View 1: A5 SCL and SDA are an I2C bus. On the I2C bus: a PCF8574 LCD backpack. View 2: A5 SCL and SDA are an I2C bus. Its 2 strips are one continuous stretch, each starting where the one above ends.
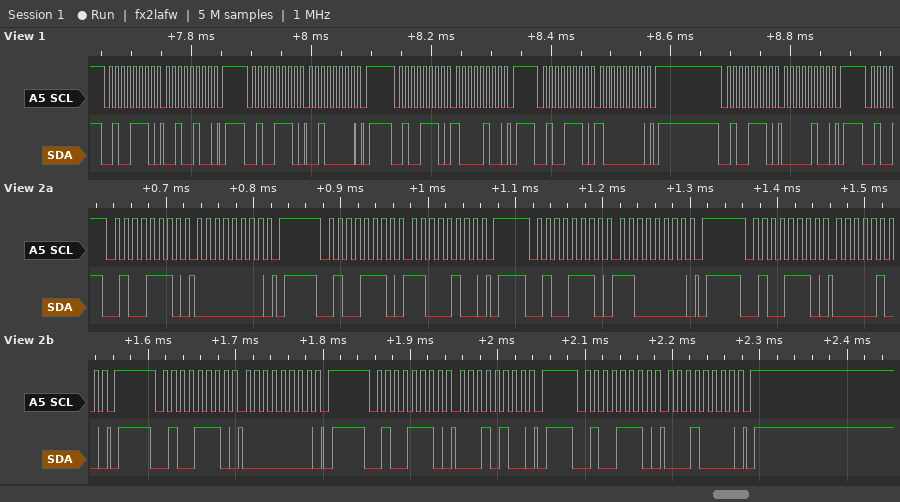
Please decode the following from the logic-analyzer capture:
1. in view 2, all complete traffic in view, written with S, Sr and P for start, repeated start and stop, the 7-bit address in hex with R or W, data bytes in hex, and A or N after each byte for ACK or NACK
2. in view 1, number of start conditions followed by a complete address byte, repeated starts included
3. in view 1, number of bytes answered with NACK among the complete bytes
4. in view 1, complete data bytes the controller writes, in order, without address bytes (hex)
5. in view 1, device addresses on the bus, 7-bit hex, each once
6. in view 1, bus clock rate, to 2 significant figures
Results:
S 27W A 00 A P S 27W A C4 A P S 27W A C0 A P S 27W A 04 A P S 27W A 00 A P S 27W A 14 A P S 27W A 10 A P
5
0
24 20 84 80 04
0x27
100 kHz
